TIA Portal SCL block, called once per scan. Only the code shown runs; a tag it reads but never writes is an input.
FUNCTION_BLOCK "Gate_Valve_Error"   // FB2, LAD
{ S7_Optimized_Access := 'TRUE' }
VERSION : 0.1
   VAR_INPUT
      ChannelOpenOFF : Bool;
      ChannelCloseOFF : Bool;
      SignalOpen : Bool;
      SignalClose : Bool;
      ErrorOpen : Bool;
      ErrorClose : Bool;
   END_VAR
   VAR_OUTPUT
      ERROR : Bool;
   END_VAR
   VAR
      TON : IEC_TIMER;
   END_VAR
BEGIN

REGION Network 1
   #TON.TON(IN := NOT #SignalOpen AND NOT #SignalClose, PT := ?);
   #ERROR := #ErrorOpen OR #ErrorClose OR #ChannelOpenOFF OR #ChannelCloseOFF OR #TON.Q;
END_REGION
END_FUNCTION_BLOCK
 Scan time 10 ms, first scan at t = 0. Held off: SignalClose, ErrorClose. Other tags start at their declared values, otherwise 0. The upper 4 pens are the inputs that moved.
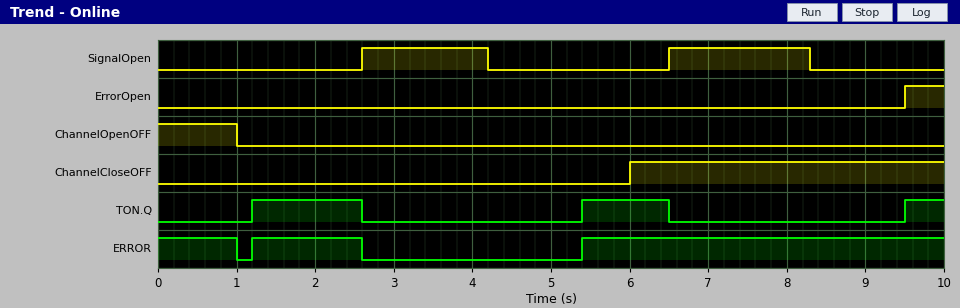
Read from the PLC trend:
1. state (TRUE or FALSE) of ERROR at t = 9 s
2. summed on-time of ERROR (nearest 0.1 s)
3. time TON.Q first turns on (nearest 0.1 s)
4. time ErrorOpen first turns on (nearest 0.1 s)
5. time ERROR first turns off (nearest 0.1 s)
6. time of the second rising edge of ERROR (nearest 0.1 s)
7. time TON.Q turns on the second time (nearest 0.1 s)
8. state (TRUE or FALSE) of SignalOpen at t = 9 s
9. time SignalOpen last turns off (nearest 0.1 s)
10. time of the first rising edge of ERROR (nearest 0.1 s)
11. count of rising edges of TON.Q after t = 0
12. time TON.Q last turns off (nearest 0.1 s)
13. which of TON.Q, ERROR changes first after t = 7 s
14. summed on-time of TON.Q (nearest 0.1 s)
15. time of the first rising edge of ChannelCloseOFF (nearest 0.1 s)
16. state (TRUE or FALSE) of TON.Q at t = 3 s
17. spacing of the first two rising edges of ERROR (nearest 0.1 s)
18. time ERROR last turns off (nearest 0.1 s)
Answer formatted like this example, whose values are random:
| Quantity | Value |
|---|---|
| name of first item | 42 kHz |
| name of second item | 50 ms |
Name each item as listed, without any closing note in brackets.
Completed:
| Quantity | Value |
|---|---|
| state (TRUE or FALSE) of ERROR at t = 9 s | TRUE |
| summed on-time of ERROR | 7.0 s |
| time TON.Q first turns on | 1.2 s |
| time ErrorOpen first turns on | 9.5 s |
| time ERROR first turns off | 1.0 s |
| time of the second rising edge of ERROR | 5.4 s |
| time TON.Q turns on the second time | 5.4 s |
| state (TRUE or FALSE) of SignalOpen at t = 9 s | FALSE |
| time SignalOpen last turns off | 8.3 s |
| time of the first rising edge of ERROR | 1.2 s |
| count of rising edges of TON.Q after t = 0 | 3 |
| time TON.Q last turns off | 6.5 s |
| which of TON.Q, ERROR changes first after t = 7 s | TON.Q |
| summed on-time of TON.Q | 3.0 s |
| time of the first rising edge of ChannelCloseOFF | 6.0 s |
| state (TRUE or FALSE) of TON.Q at t = 3 s | FALSE |
| spacing of the first two rising edges of ERROR | 4.2 s |
| time ERROR last turns off | 2.6 s |
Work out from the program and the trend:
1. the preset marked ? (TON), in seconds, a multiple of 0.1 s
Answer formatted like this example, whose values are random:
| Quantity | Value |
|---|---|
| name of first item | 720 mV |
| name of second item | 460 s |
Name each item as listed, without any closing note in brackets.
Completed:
| Quantity | Value |
|---|---|
| the preset marked ? (TON), in seconds, a multiple of 0.1 s | 1.2 s |
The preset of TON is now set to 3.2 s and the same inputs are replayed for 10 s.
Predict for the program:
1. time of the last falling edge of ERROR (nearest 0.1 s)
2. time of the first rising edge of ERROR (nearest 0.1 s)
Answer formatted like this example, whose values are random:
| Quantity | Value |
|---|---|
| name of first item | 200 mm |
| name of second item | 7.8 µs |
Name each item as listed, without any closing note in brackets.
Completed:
| Quantity | Value |
|---|---|
| time of the last falling edge of ERROR | 1.0 s |
| time of the first rising edge of ERROR | 6.0 s |
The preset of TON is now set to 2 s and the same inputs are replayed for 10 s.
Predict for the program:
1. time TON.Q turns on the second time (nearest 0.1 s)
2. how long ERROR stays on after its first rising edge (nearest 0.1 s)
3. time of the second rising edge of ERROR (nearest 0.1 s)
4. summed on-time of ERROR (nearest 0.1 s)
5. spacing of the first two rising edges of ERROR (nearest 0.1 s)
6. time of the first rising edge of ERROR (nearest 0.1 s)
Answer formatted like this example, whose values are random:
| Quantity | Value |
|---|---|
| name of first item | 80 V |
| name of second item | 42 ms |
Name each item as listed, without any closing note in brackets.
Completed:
| Quantity | Value |
|---|---|
| time TON.Q turns on the second time | 6.2 s |
| how long ERROR stays on after its first rising edge | 0.6 s |
| time of the second rising edge of ERROR | 6.0 s |
| summed on-time of ERROR | 5.6 s |
| spacing of the first two rising edges of ERROR | 4.0 s |
| time of the first rising edge of ERROR | 2.0 s |
